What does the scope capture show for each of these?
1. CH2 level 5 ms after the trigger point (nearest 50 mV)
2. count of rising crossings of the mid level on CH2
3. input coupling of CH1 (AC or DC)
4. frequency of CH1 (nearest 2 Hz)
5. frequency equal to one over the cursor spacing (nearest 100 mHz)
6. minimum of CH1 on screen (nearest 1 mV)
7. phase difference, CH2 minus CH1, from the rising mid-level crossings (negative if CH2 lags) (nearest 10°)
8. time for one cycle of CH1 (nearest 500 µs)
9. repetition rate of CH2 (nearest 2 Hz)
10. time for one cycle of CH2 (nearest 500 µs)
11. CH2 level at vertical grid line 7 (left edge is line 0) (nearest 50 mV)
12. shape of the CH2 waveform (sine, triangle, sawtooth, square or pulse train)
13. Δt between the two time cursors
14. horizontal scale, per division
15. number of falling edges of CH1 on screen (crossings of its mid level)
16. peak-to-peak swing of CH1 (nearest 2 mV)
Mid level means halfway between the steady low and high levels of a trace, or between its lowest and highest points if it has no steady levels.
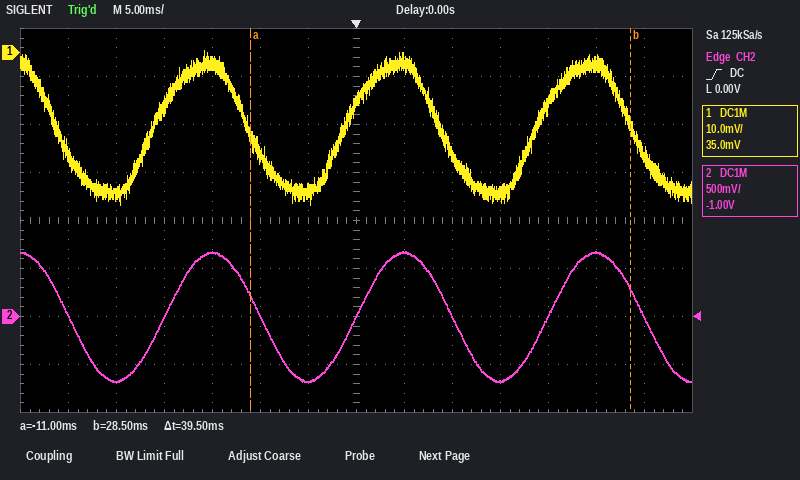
650 mV
3
DC
50 Hz
25.3 Hz
-32 mV
-20°
20.0 ms
50 Hz
20.0 ms
0 mV
sine
39.5 ms
5 ms
4
32 mV
